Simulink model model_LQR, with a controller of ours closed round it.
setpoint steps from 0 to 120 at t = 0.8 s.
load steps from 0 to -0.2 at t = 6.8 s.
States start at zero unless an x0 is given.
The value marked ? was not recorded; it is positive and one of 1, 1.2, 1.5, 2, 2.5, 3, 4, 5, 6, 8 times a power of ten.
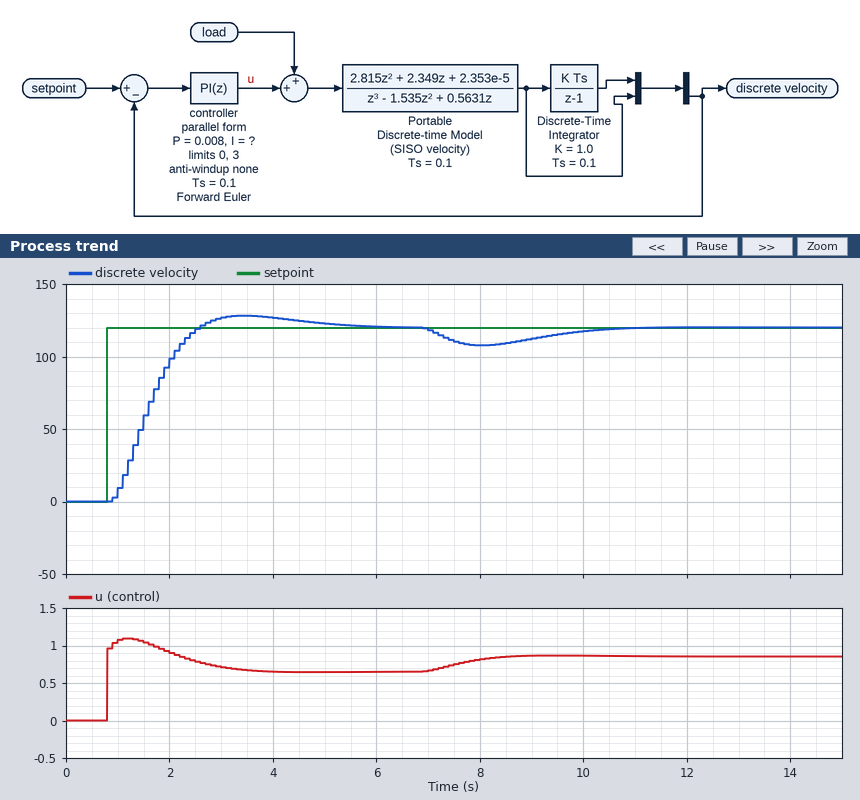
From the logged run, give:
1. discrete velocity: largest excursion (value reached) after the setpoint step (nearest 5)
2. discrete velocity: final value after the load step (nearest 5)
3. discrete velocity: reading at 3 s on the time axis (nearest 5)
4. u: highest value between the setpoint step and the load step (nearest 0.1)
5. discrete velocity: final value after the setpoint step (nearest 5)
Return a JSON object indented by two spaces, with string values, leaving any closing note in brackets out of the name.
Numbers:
{
  "discrete velocity: largest excursion (value reached) after the setpoint step": "130",
  "discrete velocity: final value after the load step": "120",
  "discrete velocity: reading at 3 s on the time axis": "125",
  "u: highest value between the setpoint step and the load step": "1.1",
  "discrete velocity: final value after the setpoint step": "120"
}
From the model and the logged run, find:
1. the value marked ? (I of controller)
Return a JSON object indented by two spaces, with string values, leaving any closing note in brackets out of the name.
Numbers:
{
  "the value marked ?": "0.008"
}
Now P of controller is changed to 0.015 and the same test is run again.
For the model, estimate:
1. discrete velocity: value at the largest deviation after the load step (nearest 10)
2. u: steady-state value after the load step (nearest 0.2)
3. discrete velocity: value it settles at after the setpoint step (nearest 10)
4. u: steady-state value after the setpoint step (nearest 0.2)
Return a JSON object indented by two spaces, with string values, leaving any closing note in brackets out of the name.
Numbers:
{
  "discrete velocity: value at the largest deviation after the load step": "110",
  "u: steady-state value after the load step": "0.8",
  "discrete velocity: value it settles at after the setpoint step": "120",
  "u: steady-state value after the setpoint step": "0.6"
}
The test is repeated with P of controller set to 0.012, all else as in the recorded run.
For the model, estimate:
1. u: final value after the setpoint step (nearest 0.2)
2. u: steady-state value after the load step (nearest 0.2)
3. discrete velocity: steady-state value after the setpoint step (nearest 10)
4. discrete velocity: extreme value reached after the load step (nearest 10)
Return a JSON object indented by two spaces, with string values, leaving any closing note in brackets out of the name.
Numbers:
{
  "u: final value after the setpoint step": "0.6",
  "u: steady-state value after the load step": "0.8",
  "discrete velocity: steady-state value after the setpoint step": "120",
  "discrete velocity: extreme value reached after the load step": "110"
}
